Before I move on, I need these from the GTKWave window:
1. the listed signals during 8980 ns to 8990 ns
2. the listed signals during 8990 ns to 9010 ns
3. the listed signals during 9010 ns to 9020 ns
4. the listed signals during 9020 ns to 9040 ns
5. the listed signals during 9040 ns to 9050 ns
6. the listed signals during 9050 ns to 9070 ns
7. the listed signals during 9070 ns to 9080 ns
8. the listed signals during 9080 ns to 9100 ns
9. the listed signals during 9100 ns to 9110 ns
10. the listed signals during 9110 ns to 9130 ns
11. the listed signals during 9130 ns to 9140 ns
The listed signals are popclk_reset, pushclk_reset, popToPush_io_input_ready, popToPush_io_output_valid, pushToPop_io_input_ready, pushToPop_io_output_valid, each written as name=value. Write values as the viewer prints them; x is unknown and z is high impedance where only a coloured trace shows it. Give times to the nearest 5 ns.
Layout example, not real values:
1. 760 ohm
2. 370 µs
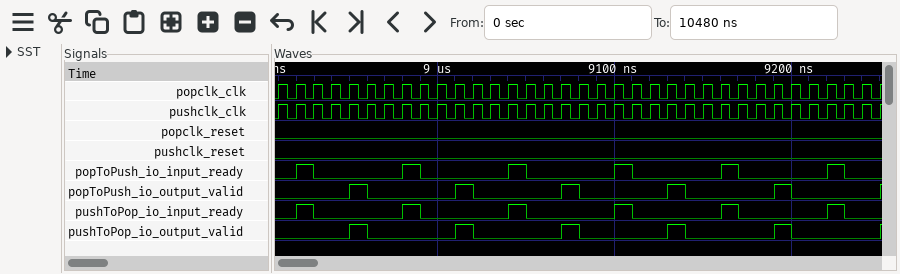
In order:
1. popclk_reset=0, pushclk_reset=0, popToPush_io_input_ready=1, popToPush_io_output_valid=0, pushToPop_io_input_ready=1, pushToPop_io_output_valid=0
2. popclk_reset=0, pushclk_reset=0, popToPush_io_input_ready=0, popToPush_io_output_valid=0, pushToPop_io_input_ready=0, pushToPop_io_output_valid=0
3. popclk_reset=0, pushclk_reset=0, popToPush_io_input_ready=0, popToPush_io_output_valid=1, pushToPop_io_input_ready=0, pushToPop_io_output_valid=1
4. popclk_reset=0, pushclk_reset=0, popToPush_io_input_ready=0, popToPush_io_output_valid=0, pushToPop_io_input_ready=0, pushToPop_io_output_valid=0
5. popclk_reset=0, pushclk_reset=0, popToPush_io_input_ready=1, popToPush_io_output_valid=0, pushToPop_io_input_ready=1, pushToPop_io_output_valid=0
6. popclk_reset=0, pushclk_reset=0, popToPush_io_input_ready=0, popToPush_io_output_valid=0, pushToPop_io_input_ready=0, pushToPop_io_output_valid=0
7. popclk_reset=0, pushclk_reset=0, popToPush_io_input_ready=0, popToPush_io_output_valid=1, pushToPop_io_input_ready=0, pushToPop_io_output_valid=1
8. popclk_reset=0, pushclk_reset=0, popToPush_io_input_ready=0, popToPush_io_output_valid=0, pushToPop_io_input_ready=0, pushToPop_io_output_valid=0
9. popclk_reset=0, pushclk_reset=0, popToPush_io_input_ready=1, popToPush_io_output_valid=0, pushToPop_io_input_ready=1, pushToPop_io_output_valid=0
10. popclk_reset=0, pushclk_reset=0, popToPush_io_input_ready=0, popToPush_io_output_valid=0, pushToPop_io_input_ready=0, pushToPop_io_output_valid=0
11. popclk_reset=0, pushclk_reset=0, popToPush_io_input_ready=0, popToPush_io_output_valid=1, pushToPop_io_input_ready=0, pushToPop_io_output_valid=1
